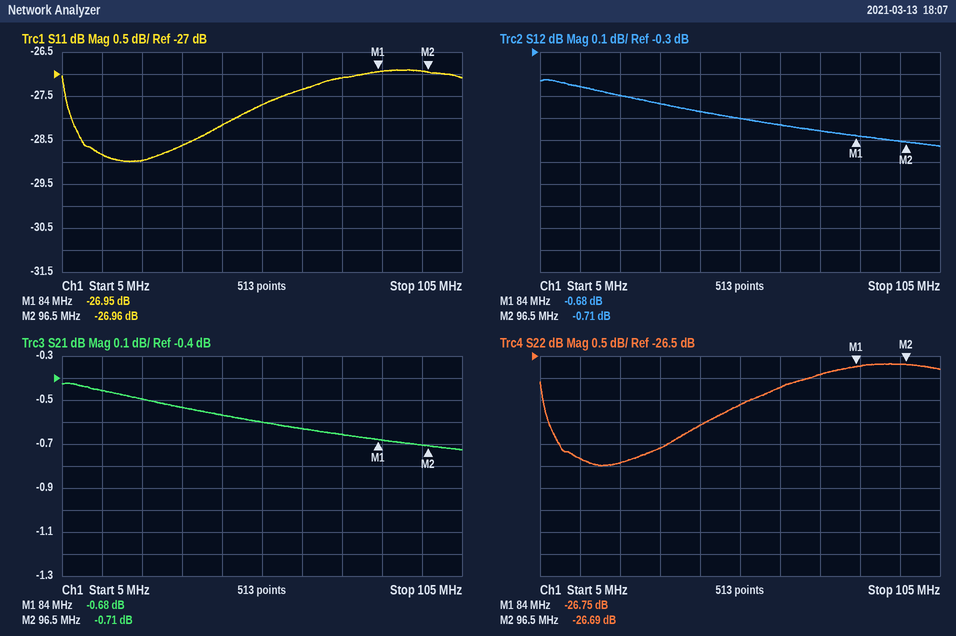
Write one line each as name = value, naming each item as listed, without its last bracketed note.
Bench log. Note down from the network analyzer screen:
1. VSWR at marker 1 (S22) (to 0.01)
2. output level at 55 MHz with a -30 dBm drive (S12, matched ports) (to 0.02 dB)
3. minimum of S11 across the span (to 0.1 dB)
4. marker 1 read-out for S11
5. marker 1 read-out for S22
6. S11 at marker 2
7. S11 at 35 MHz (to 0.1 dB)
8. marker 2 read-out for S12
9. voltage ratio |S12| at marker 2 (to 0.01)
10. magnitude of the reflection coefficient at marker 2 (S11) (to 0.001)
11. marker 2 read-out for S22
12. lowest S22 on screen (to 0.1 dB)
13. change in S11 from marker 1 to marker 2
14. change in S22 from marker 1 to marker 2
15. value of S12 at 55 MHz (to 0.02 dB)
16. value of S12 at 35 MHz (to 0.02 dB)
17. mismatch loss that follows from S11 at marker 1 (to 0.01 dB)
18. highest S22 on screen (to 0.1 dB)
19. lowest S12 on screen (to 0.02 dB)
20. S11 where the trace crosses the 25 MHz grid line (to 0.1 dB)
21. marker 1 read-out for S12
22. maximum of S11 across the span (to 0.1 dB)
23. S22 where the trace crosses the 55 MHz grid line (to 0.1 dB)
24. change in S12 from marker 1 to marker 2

VSWR at marker 1 (S22) = 1.10
output level at 55 MHz with a -30 dBm drive (S12, matched ports) = -30.60 dBm
minimum of S11 across the span = -29.0 dB
marker 1 read-out for S11 = -26.95 dB
marker 1 read-out for S22 = -26.75 dB
S11 at marker 2 = -26.96 dB
S11 at 35 MHz = -28.6 dB
marker 2 read-out for S12 = -0.71 dB
voltage ratio |S12| at marker 2 = 0.92
magnitude of the reflection coefficient at marker 2 (S11) = 0.045
marker 2 read-out for S22 = -26.69 dB
lowest S22 on screen = -29.0 dB
change in S11 from marker 1 to marker 2 = -0.01 dB
change in S22 from marker 1 to marker 2 = 0.06 dB
value of S12 at 55 MHz = -0.60 dB
value of S12 at 35 MHz = -0.54 dB
mismatch loss that follows from S11 at marker 1 = 0.01 dB
highest S22 on screen = -26.7 dB
lowest S12 on screen = -0.72 dB
S11 where the trace crosses the 25 MHz grid line = -29.0 dB
marker 1 read-out for S12 = -0.68 dB
maximum of S11 across the span = -26.9 dB
S22 where the trace crosses the 55 MHz grid line = -27.6 dB
change in S12 from marker 1 to marker 2 = -0.03 dB
